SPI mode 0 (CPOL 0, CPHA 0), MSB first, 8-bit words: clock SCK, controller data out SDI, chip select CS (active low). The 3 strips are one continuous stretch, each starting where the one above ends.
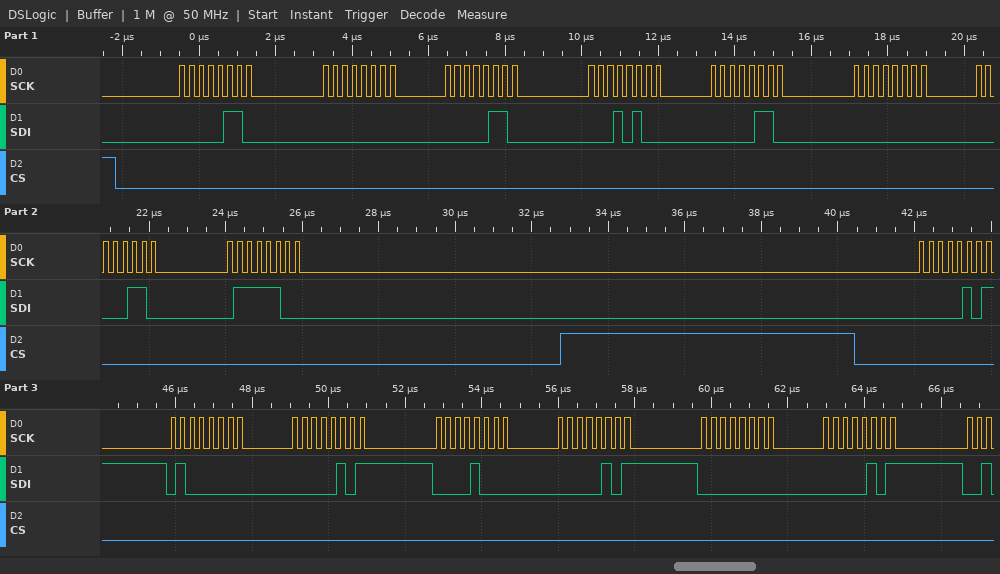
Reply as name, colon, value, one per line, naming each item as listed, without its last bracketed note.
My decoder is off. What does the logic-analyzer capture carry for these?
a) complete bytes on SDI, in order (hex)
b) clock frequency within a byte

complete bytes on SDI, in order: 06 00 06 14 06 00 06 7C 05 40 05 08 05 00 05
clock frequency within a byte: 4 MHz
